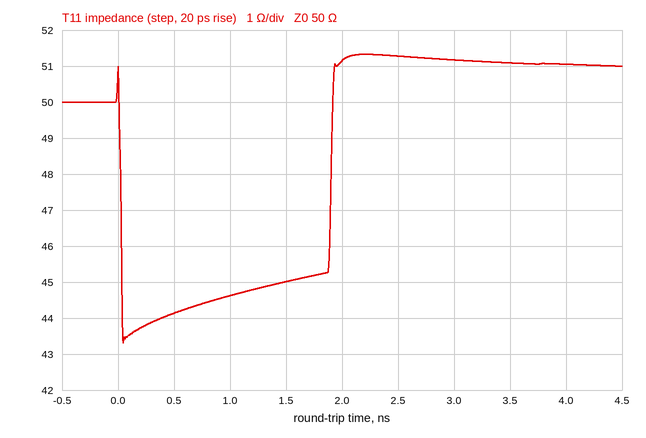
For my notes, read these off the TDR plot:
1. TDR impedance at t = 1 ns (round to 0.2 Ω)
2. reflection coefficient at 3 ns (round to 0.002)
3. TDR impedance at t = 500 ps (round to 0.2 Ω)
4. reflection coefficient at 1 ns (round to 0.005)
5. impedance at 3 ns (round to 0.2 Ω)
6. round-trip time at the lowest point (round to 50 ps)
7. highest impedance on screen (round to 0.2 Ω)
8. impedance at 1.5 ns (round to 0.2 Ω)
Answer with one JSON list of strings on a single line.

["44.6 Ω", "+0.012", "44.2 Ω", "-0.055", "51.2 Ω", "50 ps", "51.4 Ω", "45.0 Ω"]
